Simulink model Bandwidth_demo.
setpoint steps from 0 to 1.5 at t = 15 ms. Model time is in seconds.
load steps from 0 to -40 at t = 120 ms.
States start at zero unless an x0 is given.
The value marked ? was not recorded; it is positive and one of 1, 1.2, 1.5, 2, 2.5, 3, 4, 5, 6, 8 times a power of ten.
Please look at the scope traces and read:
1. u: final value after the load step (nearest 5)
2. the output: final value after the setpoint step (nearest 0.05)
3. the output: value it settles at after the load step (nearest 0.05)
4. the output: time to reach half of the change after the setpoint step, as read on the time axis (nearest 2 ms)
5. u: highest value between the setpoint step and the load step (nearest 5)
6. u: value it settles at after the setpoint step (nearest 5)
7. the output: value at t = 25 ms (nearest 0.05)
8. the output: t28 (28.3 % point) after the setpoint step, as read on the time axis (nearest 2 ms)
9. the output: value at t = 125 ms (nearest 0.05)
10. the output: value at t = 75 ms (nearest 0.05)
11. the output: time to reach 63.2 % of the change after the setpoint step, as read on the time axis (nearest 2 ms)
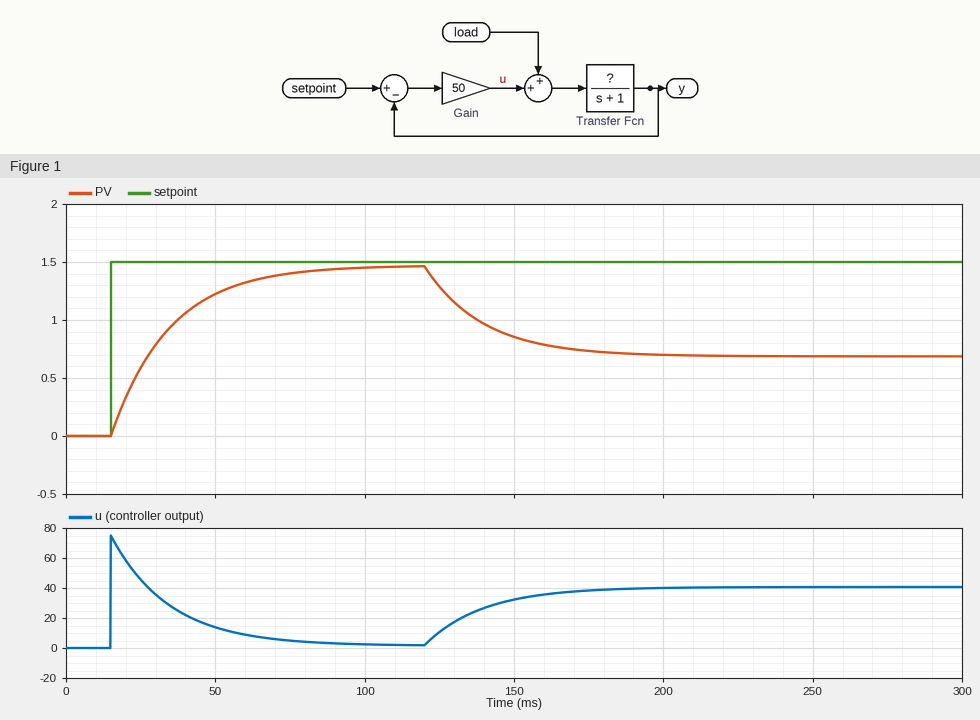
40
1.45
0.70
28 ms
75
0
0.60
22 ms
1.30
1.40
34 ms
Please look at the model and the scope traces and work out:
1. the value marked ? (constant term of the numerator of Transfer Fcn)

1
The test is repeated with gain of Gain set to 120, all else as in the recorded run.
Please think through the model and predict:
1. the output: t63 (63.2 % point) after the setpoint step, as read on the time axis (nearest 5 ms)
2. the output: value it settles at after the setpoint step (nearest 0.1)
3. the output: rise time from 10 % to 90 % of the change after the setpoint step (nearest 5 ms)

25 ms
1.5
20 ms
